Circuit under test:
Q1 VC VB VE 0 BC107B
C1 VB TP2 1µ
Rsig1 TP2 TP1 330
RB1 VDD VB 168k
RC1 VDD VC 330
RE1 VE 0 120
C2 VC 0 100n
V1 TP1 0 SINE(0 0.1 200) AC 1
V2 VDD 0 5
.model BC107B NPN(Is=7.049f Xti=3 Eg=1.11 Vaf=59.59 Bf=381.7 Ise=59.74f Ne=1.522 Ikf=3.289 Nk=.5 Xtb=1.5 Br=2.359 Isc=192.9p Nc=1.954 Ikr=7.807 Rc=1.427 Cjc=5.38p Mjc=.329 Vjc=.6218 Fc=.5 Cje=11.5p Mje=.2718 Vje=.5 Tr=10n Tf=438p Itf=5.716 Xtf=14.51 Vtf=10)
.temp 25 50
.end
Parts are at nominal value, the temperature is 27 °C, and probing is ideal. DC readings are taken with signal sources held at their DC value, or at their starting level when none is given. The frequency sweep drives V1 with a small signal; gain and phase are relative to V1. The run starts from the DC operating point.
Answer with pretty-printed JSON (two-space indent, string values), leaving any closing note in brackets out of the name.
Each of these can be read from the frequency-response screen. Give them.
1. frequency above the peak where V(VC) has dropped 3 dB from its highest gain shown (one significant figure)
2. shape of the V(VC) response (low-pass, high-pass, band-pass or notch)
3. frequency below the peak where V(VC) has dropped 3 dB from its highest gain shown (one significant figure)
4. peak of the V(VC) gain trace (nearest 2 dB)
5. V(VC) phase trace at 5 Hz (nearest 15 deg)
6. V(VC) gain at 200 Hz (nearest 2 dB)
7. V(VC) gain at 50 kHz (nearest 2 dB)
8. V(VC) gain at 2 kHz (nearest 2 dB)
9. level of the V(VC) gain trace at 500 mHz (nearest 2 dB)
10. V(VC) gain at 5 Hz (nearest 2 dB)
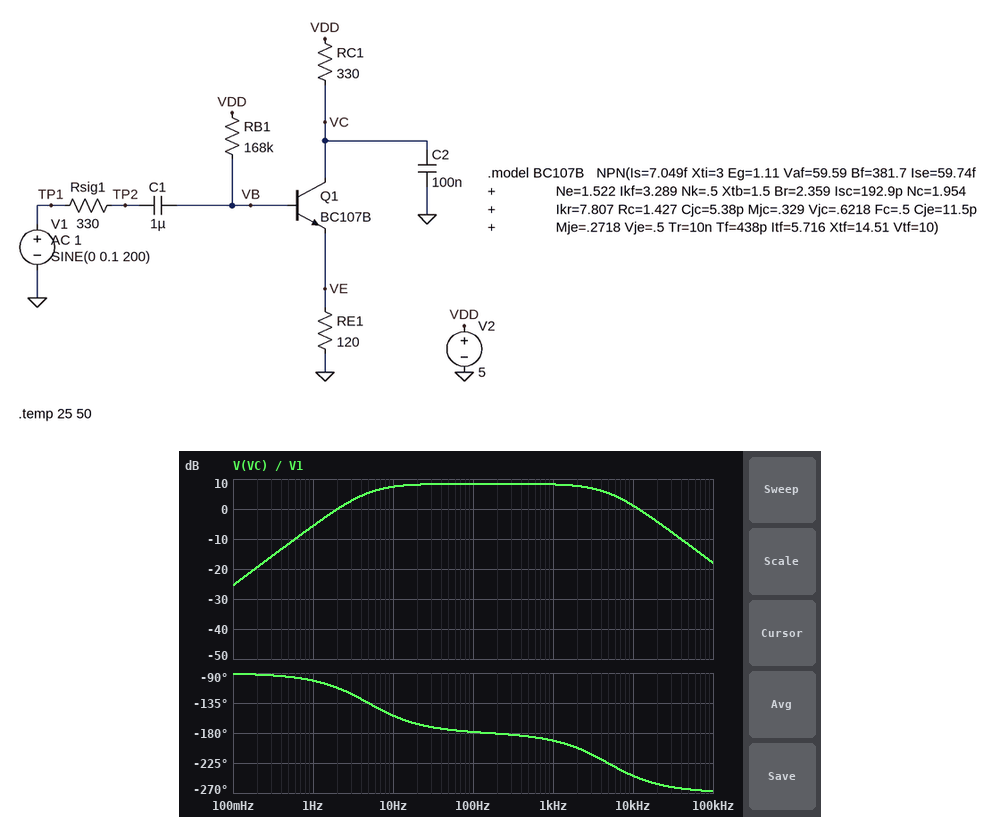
{
  "frequency above the peak where V(VC) has dropped 3 dB from its highest gain shown": "5 kHz",
  "shape of the V(VC) response": "band-pass",
  "frequency below the peak where V(VC) has dropped 3 dB from its highest gain shown": "5 Hz",
  "peak of the V(VC) gain trace": "8 dB",
  "V(VC) phase trace at 5 Hz": "-135 deg",
  "V(VC) gain at 200 Hz": "8 dB",
  "V(VC) gain at 50 kHz": "-12 dB",
  "V(VC) gain at 2 kHz": "8 dB",
  "level of the V(VC) gain trace at 500 mHz": "-12 dB",
  "V(VC) gain at 5 Hz": "6 dB"
}
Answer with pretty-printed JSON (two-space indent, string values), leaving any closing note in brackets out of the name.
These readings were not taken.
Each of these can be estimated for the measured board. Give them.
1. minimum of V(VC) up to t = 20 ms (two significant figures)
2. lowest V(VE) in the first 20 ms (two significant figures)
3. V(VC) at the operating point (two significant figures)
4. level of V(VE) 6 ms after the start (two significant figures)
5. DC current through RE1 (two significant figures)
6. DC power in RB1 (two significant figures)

{
  "minimum of V(VC) up to t = 20 ms": "2.6 V",
  "lowest V(VE) in the first 20 ms": "680 mV",
  "V(VC) at the operating point": "2.9 V",
  "level of V(VE) 6 ms after the start": "870 mV",
  "DC current through RE1": "6.5 mA",
  "DC power in RB1": "73 µW"
}
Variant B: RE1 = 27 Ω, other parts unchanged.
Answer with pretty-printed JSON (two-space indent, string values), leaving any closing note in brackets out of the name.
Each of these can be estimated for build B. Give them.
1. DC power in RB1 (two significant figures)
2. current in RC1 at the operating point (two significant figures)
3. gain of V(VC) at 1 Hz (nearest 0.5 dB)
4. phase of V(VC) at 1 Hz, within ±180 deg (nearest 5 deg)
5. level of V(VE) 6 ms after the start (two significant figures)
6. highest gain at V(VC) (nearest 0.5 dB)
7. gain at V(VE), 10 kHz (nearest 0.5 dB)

{
  "DC power in RB1": "99 µW",
  "current in RC1 at the operating point": "7.6 mA",
  "gain of V(VC) at 1 Hz": "-4.0 dB",
  "phase of V(VC) at 1 Hz, within ±180 deg": "-95 deg",
  "level of V(VE) 6 ms after the start": "290 mV",
  "highest gain at V(VC)": "20.5 dB",
  "gain at V(VE), 10 kHz": "-1.5 dB"
}
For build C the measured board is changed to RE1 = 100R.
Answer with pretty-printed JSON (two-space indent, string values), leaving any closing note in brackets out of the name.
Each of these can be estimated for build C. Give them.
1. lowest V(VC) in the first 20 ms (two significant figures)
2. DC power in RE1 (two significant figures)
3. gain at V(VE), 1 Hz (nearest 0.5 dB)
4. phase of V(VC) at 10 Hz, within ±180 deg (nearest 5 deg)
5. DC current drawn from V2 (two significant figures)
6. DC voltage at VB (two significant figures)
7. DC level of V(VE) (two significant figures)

{
  "lowest V(VC) in the first 20 ms": "2.5 V",
  "DC power in RE1": "4.5 mW",
  "gain at V(VE), 1 Hz": "-15.5 dB",
  "phase of V(VC) at 10 Hz, within ±180 deg": "-150 deg",
  "DC current drawn from V2": "6.7 mA",
  "DC voltage at VB": "1.4 V",
  "DC level of V(VE)": "670 mV"
}
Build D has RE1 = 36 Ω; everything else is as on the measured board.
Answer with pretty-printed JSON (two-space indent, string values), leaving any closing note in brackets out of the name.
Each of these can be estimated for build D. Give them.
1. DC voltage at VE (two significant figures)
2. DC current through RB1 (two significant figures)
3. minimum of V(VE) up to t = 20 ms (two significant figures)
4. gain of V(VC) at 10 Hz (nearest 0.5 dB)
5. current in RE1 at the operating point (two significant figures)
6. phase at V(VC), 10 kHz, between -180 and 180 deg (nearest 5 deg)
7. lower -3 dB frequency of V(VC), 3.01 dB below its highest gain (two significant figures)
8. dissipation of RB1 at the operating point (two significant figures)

{
  "DC voltage at VE": "270 mV",
  "DC current through RB1": "24 µA",
  "minimum of V(VE) up to t = 20 ms": "180 mV",
  "gain of V(VC) at 10 Hz": "14.0 dB",
  "current in RE1 at the operating point": "7.5 mA",
  "phase at V(VC), 10 kHz, between -180 and 180 deg": "115 deg",
  "lower -3 dB frequency of V(VC), 3.01 dB below its highest gain": "13 Hz",
  "dissipation of RB1 at the operating point": "96 µW"
}
